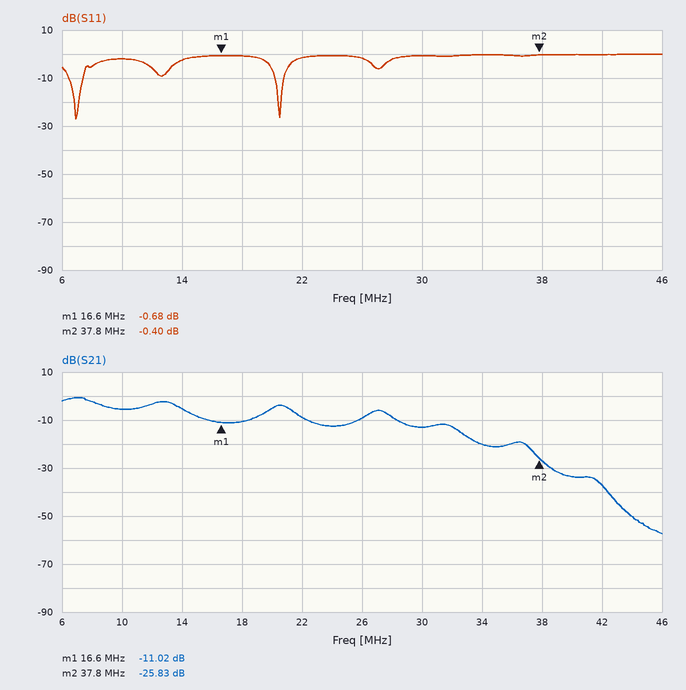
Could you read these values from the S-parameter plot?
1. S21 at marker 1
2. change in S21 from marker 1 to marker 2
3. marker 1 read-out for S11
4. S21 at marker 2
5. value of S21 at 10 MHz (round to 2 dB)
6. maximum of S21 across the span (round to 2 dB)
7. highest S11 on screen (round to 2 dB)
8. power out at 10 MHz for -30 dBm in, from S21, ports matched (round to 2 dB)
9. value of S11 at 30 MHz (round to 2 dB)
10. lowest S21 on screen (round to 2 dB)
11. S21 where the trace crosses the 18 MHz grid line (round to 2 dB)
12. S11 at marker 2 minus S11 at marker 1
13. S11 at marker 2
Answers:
-11.02 dB
-14.81 dB
-0.68 dB
-25.83 dB
-6 dB
0 dB
0 dB
-36 dBm
0 dB
-58 dB
-10 dB
0.28 dB
-0.40 dB
